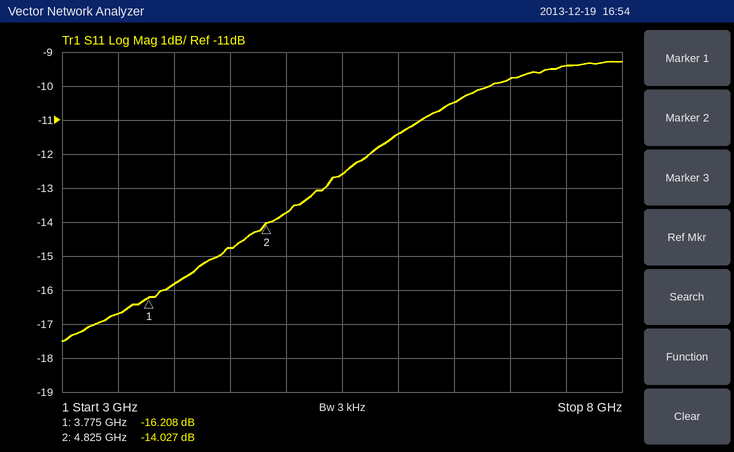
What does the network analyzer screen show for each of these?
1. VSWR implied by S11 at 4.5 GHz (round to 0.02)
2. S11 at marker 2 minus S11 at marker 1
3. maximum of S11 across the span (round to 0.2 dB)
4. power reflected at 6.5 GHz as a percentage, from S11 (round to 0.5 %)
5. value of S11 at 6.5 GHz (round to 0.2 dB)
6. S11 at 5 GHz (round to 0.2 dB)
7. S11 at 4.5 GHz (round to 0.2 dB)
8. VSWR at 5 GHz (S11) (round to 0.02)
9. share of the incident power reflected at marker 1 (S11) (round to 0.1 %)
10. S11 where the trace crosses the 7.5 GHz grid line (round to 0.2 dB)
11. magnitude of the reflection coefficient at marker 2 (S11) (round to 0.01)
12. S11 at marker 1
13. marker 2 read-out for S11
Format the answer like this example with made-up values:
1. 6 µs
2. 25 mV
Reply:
1. 1.44
2. 2.181 dB
3. -9.2 dB
4. 9.0 %
5. -10.4 dB
6. -13.8 dB
7. -14.8 dB
8. 1.52
9. 2.4 %
10. -9.4 dB
11. 0.20
12. -16.208 dB
13. -14.027 dB
